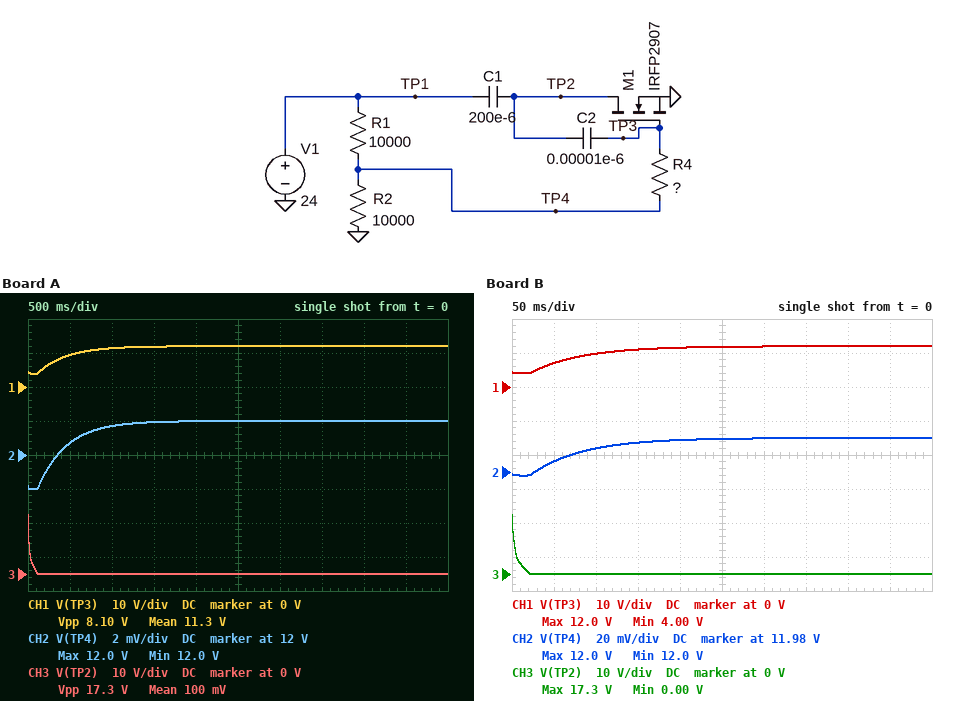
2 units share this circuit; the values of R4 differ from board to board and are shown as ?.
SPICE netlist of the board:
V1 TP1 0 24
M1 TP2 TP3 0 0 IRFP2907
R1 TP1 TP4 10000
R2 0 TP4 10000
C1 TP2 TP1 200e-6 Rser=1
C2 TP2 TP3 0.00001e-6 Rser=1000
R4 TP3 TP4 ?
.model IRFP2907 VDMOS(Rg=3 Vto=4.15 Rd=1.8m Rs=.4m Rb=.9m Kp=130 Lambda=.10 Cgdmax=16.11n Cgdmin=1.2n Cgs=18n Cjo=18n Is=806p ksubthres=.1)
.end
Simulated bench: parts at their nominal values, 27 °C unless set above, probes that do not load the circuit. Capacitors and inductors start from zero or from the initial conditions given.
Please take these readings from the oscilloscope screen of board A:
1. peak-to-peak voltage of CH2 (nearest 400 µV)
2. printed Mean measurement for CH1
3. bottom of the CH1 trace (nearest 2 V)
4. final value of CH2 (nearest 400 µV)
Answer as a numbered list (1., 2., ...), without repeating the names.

1. 4.0 mV
2. 11.3 V
3. 4 V
4. 12.0000 V
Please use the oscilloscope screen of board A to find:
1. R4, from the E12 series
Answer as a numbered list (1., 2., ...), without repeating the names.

1. 10 MΩ
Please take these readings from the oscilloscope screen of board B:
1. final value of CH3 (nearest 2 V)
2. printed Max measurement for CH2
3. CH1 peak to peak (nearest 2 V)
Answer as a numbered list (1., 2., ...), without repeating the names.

1. 0 V
2. 12.0 V
3. 8 V
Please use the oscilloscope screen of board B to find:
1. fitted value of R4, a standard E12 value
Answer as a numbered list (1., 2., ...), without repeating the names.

1. 1.8 MΩ
